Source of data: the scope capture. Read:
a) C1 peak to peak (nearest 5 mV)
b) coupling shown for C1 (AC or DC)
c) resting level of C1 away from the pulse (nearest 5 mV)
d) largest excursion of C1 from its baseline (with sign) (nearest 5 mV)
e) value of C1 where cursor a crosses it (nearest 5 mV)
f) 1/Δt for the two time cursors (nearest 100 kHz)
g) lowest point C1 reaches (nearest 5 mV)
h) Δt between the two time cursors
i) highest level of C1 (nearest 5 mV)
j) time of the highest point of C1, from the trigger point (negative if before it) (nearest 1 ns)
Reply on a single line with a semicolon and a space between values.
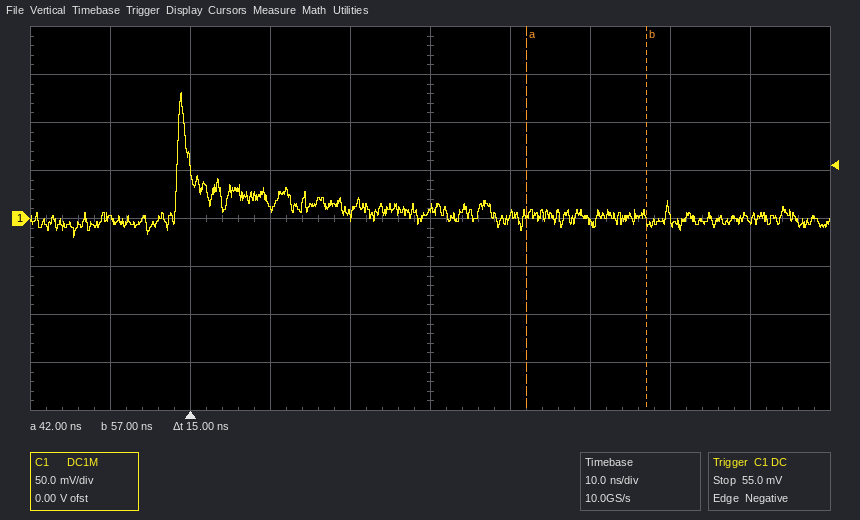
150 mV; DC; 0 mV; +130 mV; 5 mV; 66.7 MHz; -20 mV; 15 ns; 130 mV; -1 ns
